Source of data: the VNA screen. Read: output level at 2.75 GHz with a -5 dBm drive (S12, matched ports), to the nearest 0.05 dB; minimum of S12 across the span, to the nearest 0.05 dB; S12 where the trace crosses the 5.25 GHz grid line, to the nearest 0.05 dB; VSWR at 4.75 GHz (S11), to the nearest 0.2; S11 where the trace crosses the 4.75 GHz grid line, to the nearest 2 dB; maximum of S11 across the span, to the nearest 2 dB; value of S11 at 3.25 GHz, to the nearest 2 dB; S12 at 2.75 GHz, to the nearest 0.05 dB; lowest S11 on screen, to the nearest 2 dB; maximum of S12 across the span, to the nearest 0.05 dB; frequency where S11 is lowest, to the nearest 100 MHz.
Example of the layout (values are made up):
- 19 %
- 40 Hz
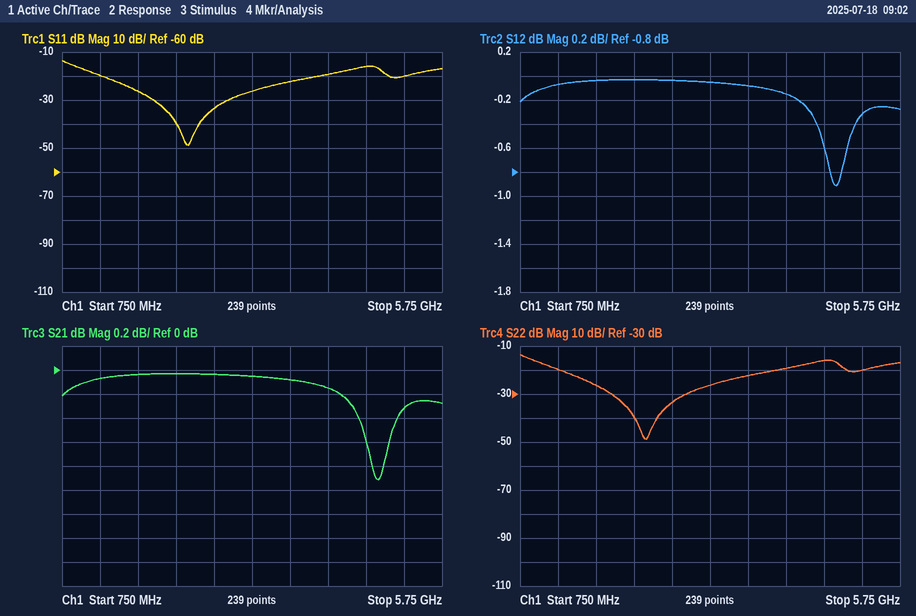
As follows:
- -5.05 dBm
- -0.90 dB
- -0.30 dB
- 1.4
- -16 dB
- -14 dB
- -26 dB
- -0.05 dB
- -48 dB
- -0.05 dB
- 2.4 GHz
